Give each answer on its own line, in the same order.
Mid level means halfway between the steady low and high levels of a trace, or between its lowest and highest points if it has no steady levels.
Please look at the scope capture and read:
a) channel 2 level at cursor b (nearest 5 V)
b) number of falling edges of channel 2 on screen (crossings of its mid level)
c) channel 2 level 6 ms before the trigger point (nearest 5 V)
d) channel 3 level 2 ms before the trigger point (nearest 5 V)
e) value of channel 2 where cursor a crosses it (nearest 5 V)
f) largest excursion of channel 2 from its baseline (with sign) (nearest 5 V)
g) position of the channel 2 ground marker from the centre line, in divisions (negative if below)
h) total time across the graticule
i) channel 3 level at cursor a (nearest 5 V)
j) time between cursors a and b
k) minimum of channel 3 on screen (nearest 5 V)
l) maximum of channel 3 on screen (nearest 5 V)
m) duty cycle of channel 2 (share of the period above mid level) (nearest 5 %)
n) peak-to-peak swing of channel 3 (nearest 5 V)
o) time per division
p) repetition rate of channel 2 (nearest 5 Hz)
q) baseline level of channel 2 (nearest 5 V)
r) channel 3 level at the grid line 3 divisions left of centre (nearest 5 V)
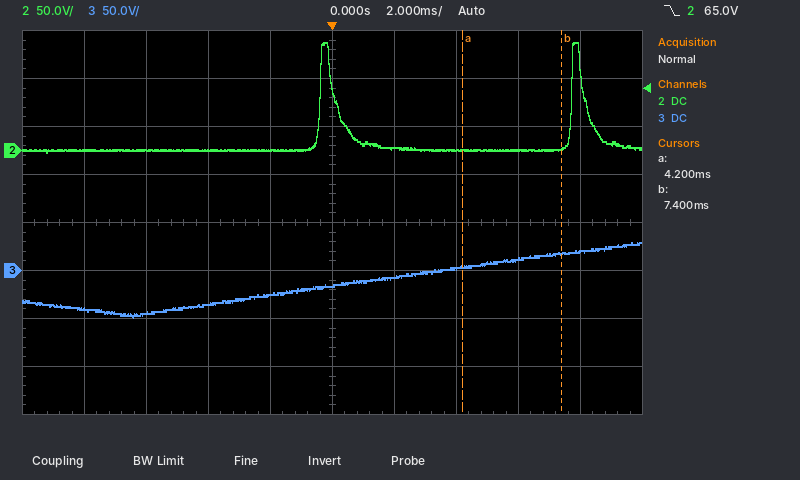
0 V
2
0 V
-25 V
0 V
+110 V
+1.5 div
20 ms
5 V
3.2 ms
-50 V
30 V
5 %
80 V
2 ms
125 Hz
0 V
-45 V
